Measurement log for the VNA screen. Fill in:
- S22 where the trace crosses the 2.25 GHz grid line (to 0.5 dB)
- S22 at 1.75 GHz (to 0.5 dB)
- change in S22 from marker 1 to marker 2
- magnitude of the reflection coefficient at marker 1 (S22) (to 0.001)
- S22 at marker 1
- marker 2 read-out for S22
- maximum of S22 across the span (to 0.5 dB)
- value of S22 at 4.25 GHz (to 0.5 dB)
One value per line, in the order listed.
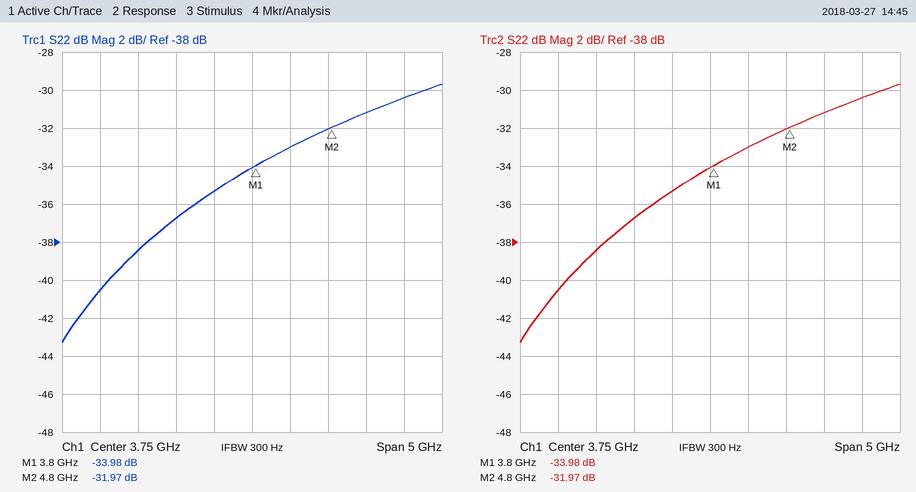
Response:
-38.5 dB
-40.5 dB
2.01 dB
0.020
-33.98 dB
-31.97 dB
-29.5 dB
-33.0 dB
